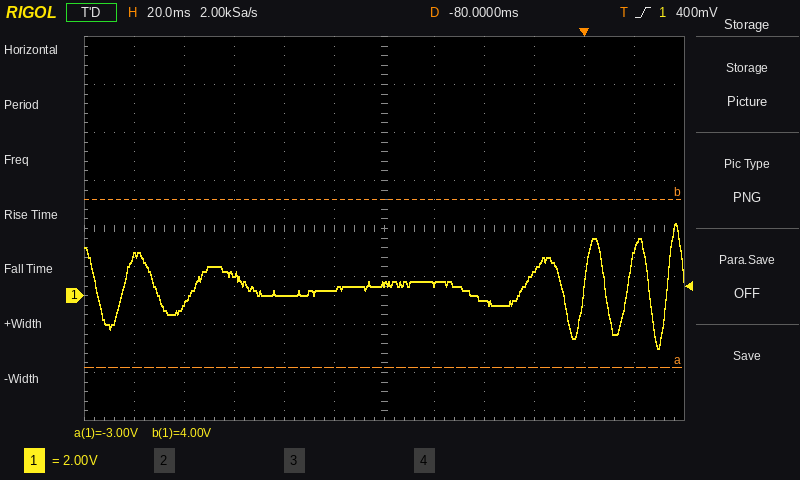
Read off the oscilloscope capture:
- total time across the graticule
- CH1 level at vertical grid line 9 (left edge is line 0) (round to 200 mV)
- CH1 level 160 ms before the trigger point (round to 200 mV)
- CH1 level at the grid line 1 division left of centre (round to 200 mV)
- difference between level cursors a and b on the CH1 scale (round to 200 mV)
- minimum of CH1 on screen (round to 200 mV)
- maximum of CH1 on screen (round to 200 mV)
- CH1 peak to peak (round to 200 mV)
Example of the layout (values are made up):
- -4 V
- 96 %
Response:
- 240 ms
- 1.0 V
- -400 mV
- 200 mV
- 7.0 V
- -2.2 V
- 3.0 V
- 5.2 V
